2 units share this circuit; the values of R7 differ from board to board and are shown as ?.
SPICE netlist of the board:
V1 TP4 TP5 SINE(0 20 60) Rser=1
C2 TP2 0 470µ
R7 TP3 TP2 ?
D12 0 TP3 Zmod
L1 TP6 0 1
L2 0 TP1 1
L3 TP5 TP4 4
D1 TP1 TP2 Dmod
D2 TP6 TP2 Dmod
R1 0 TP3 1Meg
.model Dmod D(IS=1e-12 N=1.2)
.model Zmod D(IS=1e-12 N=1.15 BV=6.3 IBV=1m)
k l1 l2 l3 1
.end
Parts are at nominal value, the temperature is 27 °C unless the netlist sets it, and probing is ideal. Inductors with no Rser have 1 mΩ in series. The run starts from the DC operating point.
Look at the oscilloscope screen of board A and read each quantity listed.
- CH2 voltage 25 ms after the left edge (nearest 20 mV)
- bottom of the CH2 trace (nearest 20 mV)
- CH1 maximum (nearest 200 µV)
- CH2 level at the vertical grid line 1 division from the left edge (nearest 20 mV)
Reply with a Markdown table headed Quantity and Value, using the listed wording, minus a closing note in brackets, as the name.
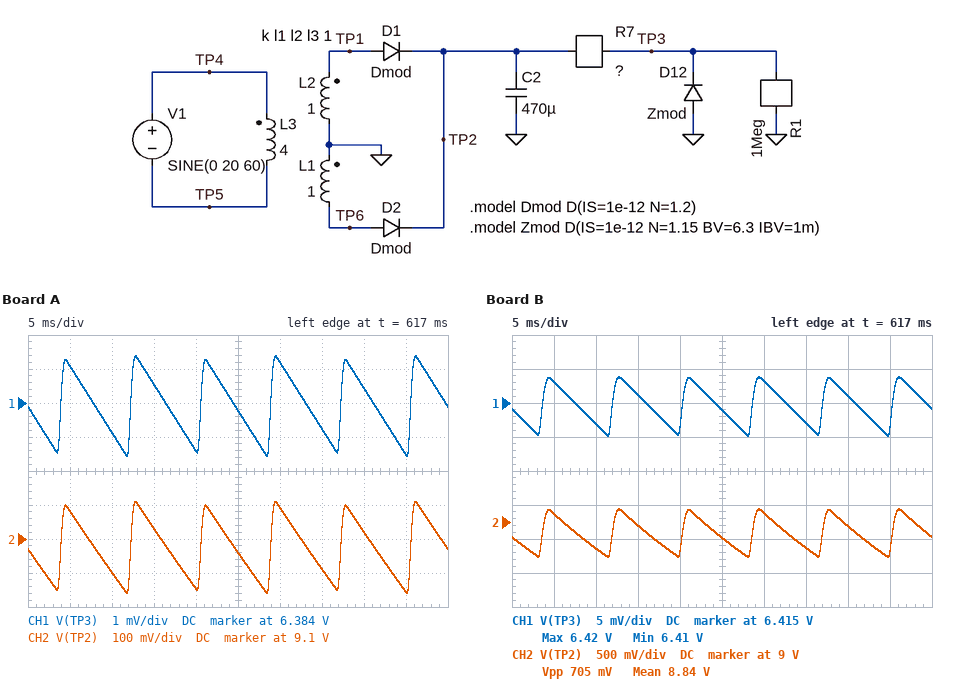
| Quantity | Value |
|---|---|
| CH2 voltage 25 ms after the left edge | 9.06 V |
| bottom of the CH2 trace | 8.94 V |
| CH1 maximum | 6.3854 V |
| CH2 level at the vertical grid line 1 division from the left edge | 9.18 V |
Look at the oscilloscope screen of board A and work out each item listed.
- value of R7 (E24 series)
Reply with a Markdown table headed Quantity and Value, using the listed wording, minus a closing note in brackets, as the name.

| Quantity | Value |
|---|---|
| value of R7 | 160 Ω |
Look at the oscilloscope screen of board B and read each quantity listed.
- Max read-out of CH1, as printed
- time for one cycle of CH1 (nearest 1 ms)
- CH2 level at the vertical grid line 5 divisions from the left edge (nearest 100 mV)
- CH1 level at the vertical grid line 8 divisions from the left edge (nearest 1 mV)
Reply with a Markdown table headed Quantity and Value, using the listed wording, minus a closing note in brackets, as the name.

| Quantity | Value |
|---|---|
| Max read-out of CH1, as printed | 6.42 V |
| time for one cycle of CH1 | 8 ms |
| CH2 level at the vertical grid line 5 divisions from the left edge | 8.8 V |
| CH1 level at the vertical grid line 8 divisions from the left edge | 6.416 V |
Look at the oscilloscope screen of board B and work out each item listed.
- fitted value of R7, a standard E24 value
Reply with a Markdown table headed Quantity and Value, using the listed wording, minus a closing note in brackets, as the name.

| Quantity | Value |
|---|---|
| fitted value of R7, a standard E24 value | 51 Ω |
